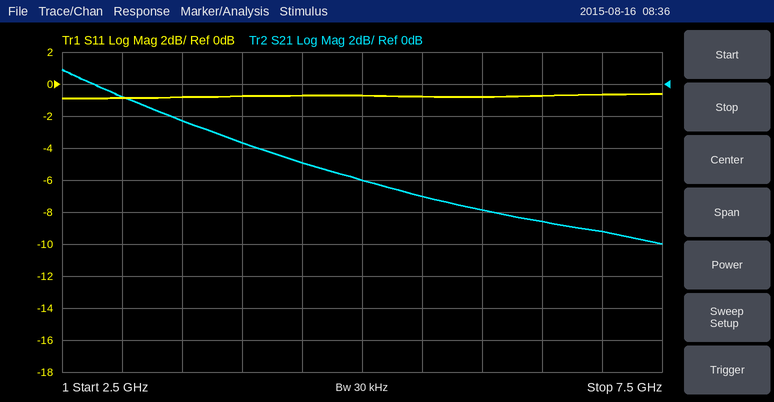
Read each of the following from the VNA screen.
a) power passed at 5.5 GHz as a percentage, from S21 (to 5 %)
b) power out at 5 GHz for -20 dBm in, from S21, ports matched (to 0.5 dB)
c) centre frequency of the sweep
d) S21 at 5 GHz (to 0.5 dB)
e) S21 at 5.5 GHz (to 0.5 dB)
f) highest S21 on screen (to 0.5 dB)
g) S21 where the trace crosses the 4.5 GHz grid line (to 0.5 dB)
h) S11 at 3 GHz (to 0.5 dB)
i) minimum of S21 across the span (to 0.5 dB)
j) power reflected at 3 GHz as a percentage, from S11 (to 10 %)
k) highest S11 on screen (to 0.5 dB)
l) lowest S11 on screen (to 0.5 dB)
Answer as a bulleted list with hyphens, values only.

- 20 %
- -26.0 dBm
- 5 GHz
- -6.0 dB
- -7.0 dB
- 1.0 dB
- -5.0 dB
- -1.0 dB
- -10.0 dB
- 80 %
- -0.5 dB
- -1.0 dB
